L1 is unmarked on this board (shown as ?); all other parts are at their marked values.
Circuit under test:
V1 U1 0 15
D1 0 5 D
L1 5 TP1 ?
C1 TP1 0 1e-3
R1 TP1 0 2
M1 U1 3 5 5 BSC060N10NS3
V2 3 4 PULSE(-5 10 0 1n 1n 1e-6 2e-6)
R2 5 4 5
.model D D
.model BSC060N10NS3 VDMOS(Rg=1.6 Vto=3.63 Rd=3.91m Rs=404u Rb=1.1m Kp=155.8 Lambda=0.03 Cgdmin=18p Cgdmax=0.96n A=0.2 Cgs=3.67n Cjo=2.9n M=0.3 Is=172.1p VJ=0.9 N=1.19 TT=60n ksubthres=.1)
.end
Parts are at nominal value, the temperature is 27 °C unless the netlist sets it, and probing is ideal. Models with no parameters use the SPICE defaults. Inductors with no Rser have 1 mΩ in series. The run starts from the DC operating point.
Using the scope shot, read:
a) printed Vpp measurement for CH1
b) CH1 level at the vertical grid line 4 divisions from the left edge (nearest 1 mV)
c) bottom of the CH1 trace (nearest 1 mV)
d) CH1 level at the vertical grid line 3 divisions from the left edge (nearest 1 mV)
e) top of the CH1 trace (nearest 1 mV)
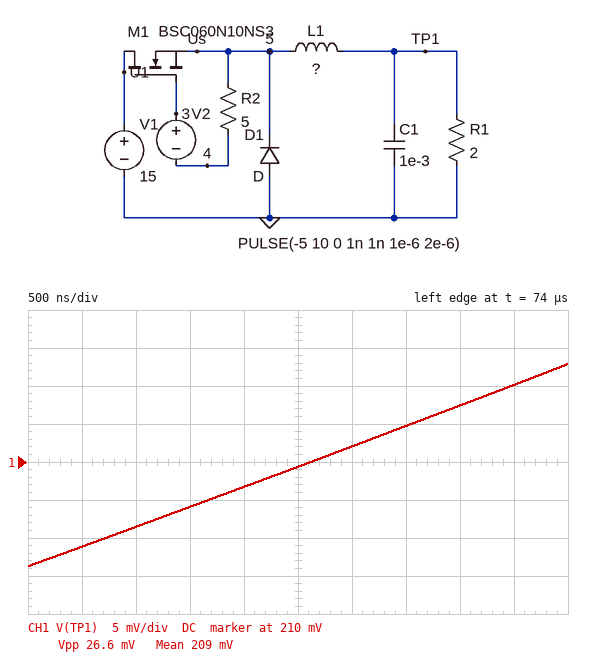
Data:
26.6 mV
207 mV
196 mV
204 mV
223 mV
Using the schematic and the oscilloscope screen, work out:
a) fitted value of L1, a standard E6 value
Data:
100 µH
